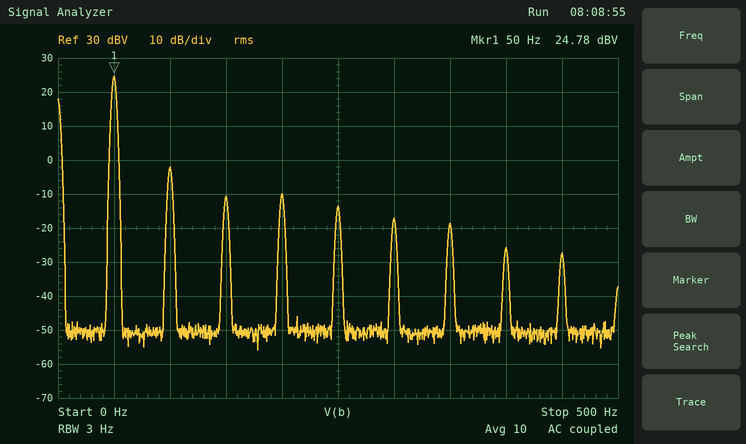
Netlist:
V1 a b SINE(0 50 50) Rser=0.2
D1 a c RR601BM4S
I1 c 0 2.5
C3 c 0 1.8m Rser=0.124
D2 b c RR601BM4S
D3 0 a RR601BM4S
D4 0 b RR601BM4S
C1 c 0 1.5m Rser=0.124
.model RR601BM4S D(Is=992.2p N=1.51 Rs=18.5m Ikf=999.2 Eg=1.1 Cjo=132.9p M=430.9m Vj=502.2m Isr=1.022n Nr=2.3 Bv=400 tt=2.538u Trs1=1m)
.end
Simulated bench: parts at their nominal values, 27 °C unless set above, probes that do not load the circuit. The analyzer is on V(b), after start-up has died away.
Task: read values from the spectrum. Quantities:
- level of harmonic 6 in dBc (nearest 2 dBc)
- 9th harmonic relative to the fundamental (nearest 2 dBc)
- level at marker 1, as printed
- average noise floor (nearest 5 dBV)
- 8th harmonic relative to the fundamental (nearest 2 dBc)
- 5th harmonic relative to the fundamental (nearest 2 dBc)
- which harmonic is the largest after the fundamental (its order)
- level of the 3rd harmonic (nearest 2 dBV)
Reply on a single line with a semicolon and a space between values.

-42 dBc; -52 dBc; 24.78 dBV; -50 dBV; -50 dBc; -38 dBc; 2; -10 dBV
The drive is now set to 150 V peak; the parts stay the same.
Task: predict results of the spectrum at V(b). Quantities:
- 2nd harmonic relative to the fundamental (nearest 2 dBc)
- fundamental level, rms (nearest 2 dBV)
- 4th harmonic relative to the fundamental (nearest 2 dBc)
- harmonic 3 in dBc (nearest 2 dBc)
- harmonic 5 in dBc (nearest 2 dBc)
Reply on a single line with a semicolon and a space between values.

-36 dBc; 34 dBV; -42 dBc; -44 dBc; -46 dBc
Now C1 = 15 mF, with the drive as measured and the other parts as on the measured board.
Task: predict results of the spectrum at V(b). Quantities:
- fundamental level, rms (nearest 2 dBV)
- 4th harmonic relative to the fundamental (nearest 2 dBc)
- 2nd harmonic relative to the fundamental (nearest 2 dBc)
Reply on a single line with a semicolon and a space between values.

24 dBV; -42 dBc; -38 dBc
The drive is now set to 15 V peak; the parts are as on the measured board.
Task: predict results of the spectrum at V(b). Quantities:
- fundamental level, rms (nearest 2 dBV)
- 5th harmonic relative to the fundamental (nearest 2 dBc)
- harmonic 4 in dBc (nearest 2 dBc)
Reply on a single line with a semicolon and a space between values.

14 dBV; -36 dBc; -28 dBc
